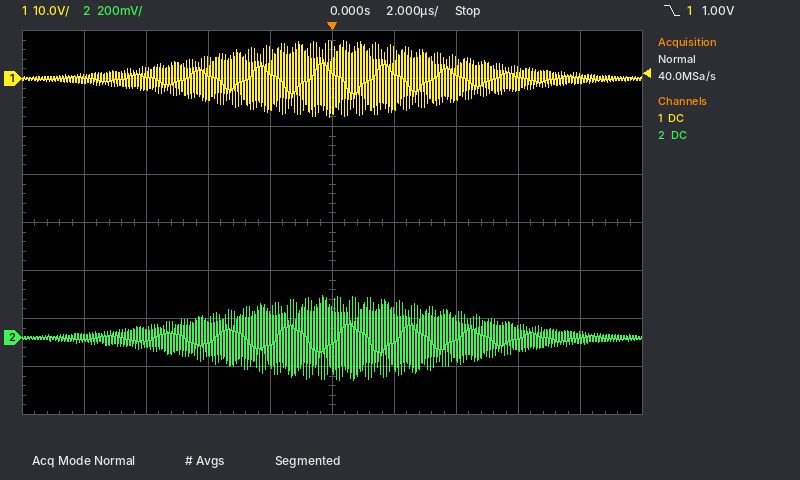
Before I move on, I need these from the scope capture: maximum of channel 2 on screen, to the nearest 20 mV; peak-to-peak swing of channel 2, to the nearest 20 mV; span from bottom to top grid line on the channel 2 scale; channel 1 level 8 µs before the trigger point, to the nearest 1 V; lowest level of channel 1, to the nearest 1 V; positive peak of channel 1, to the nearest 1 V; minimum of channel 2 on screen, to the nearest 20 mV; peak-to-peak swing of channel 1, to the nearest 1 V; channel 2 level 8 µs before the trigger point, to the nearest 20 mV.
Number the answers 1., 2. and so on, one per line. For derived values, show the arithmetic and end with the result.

1. 180 mV
2. 180 mV − (-180 mV) = 360 mV
3. 1.6 V
4. 0 V
5. -8 V
6. 8 V
7. -180 mV
8. 8 V − (-8 V) = 16 V
9. 0 mV
